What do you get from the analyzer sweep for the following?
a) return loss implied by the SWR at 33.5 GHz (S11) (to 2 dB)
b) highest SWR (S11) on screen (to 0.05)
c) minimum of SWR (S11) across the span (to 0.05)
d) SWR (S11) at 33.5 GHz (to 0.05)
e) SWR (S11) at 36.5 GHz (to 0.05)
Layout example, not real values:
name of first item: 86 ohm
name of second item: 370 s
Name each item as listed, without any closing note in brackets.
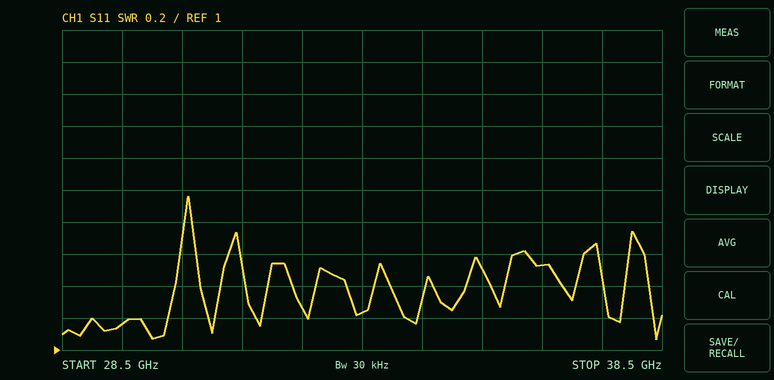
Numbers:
return loss implied by the SWR at 33.5 GHz (S11): 20 dB
highest SWR (S11) on screen: 1.95
minimum of SWR (S11) across the span: 1.05
SWR (S11) at 33.5 GHz: 1.25
SWR (S11) at 36.5 GHz: 1.55
